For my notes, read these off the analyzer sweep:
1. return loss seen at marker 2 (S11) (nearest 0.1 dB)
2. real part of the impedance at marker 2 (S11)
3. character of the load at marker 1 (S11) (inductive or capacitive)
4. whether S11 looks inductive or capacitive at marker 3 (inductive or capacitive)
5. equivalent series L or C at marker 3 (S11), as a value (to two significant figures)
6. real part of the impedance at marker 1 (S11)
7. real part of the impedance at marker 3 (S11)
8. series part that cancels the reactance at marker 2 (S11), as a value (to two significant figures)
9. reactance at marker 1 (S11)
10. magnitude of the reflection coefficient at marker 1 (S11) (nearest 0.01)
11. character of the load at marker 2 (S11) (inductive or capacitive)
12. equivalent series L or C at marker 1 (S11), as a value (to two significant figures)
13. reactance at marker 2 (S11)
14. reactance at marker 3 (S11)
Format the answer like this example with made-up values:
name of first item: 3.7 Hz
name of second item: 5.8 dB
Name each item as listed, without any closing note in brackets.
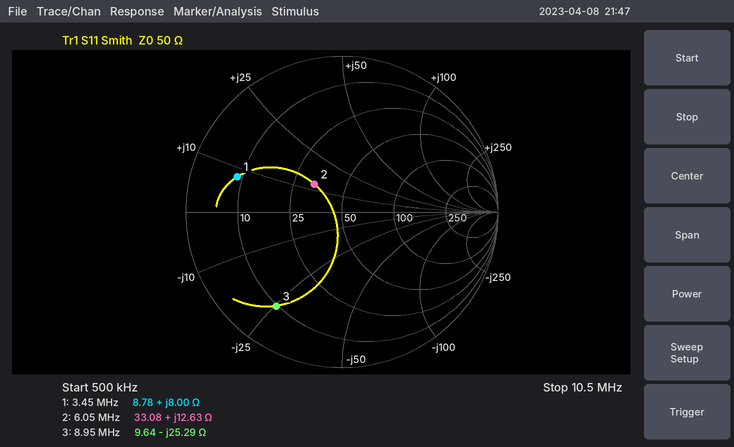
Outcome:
return loss seen at marker 2 (S11): 12.0 dB
real part of the impedance at marker 2: 33.08 Ω
character of the load at marker 1 (S11): inductive
whether S11 looks inductive or capacitive at marker 3: capacitive
equivalent series L or C at marker 3 (S11), as a value: 700 pF
real part of the impedance at marker 1: 8.78 Ω
real part of the impedance at marker 3: 9.64 Ω
series part that cancels the reactance at marker 2 (S11), as a value: 2.1 nF
reactance at marker 1: +8.00 Ω
magnitude of the reflection coefficient at marker 1 (S11): 0.71
character of the load at marker 2 (S11): inductive
equivalent series L or C at marker 1 (S11), as a value: 370 nH
reactance at marker 2: +12.63 Ω
reactance at marker 3: -25.29 Ω
